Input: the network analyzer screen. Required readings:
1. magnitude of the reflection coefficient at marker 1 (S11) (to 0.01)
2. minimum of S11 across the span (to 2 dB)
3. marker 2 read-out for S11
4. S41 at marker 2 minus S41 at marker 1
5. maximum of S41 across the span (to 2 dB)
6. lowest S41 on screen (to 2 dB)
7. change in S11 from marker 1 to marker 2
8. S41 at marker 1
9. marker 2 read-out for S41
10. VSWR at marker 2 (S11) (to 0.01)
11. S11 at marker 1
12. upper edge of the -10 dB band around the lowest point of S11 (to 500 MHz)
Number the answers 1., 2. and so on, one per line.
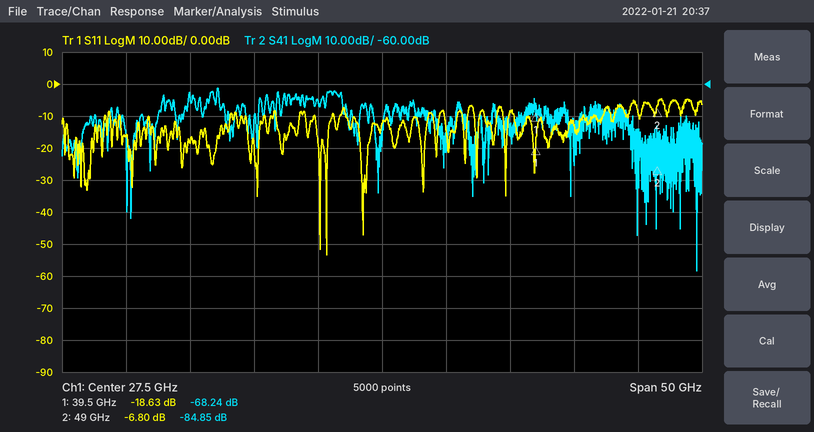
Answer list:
1. 0.12
2. -54 dB
3. -6.80 dB
4. -16.61 dB
5. -62 dB
6. -118 dB
7. 11.83 dB
8. -68.24 dB
9. -84.85 dB
10. 2.68
11. -18.63 dB
12. 23.5 GHz
